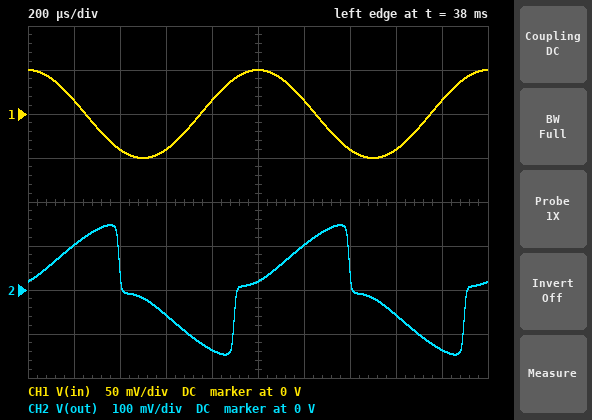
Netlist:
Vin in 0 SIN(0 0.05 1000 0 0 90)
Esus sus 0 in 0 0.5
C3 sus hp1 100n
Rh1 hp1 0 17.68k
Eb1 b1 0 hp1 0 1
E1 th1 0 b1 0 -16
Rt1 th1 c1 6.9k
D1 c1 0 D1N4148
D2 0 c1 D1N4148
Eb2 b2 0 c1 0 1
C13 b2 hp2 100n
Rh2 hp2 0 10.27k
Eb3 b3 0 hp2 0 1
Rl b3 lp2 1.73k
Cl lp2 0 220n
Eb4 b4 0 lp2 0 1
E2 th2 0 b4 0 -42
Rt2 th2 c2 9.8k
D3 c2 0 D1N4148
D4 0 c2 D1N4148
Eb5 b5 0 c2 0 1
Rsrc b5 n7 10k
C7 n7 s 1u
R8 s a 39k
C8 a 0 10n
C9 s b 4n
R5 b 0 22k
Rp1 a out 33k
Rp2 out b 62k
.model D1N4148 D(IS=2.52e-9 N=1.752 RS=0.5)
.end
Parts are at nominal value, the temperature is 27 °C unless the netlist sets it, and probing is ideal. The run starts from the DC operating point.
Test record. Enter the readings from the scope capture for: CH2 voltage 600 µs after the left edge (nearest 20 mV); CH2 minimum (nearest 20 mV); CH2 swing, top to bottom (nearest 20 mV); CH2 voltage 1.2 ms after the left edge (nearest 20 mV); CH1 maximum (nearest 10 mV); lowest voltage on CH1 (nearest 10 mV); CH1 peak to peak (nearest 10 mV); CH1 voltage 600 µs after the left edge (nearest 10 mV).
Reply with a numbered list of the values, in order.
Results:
1. -60 mV
2. -140 mV
3. 300 mV
4. 100 mV
5. 50 mV
6. -50 mV
7. 100 mV
8. -40 mV
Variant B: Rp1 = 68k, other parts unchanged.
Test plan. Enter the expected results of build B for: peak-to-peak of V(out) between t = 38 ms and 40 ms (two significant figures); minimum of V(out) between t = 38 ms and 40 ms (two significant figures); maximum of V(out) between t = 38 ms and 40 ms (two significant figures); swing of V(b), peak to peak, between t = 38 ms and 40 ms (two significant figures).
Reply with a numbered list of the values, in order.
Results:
1. 230 mV
2. -110 mV
3. 110 mV
4. 800 mV
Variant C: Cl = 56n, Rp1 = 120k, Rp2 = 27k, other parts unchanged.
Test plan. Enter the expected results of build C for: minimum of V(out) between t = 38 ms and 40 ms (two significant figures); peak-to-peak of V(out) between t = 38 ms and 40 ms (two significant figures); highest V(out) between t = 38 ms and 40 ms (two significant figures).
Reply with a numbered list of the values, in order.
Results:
1. -340 mV
2. 680 mV
3. 340 mV
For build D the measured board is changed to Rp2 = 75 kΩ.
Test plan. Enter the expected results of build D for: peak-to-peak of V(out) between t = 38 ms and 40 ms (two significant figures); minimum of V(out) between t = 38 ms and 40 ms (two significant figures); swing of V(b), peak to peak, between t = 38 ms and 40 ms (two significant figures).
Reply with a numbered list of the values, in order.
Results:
1. 310 mV
2. -150 mV
3. 780 mV
